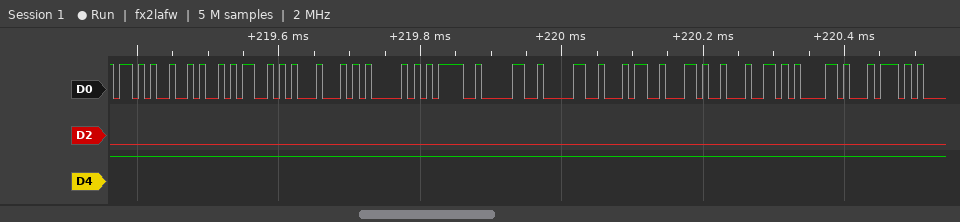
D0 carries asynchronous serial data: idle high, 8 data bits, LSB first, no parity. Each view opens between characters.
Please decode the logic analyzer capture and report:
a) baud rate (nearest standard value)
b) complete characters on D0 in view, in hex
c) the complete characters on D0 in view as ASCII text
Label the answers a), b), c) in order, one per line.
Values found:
a) 115200 baud
b) 2B, 4A, 53, 44, 41, 3D, 30, 30, 34, 2C, 64, 61, 74
c) "+JSDA=004,dat"
